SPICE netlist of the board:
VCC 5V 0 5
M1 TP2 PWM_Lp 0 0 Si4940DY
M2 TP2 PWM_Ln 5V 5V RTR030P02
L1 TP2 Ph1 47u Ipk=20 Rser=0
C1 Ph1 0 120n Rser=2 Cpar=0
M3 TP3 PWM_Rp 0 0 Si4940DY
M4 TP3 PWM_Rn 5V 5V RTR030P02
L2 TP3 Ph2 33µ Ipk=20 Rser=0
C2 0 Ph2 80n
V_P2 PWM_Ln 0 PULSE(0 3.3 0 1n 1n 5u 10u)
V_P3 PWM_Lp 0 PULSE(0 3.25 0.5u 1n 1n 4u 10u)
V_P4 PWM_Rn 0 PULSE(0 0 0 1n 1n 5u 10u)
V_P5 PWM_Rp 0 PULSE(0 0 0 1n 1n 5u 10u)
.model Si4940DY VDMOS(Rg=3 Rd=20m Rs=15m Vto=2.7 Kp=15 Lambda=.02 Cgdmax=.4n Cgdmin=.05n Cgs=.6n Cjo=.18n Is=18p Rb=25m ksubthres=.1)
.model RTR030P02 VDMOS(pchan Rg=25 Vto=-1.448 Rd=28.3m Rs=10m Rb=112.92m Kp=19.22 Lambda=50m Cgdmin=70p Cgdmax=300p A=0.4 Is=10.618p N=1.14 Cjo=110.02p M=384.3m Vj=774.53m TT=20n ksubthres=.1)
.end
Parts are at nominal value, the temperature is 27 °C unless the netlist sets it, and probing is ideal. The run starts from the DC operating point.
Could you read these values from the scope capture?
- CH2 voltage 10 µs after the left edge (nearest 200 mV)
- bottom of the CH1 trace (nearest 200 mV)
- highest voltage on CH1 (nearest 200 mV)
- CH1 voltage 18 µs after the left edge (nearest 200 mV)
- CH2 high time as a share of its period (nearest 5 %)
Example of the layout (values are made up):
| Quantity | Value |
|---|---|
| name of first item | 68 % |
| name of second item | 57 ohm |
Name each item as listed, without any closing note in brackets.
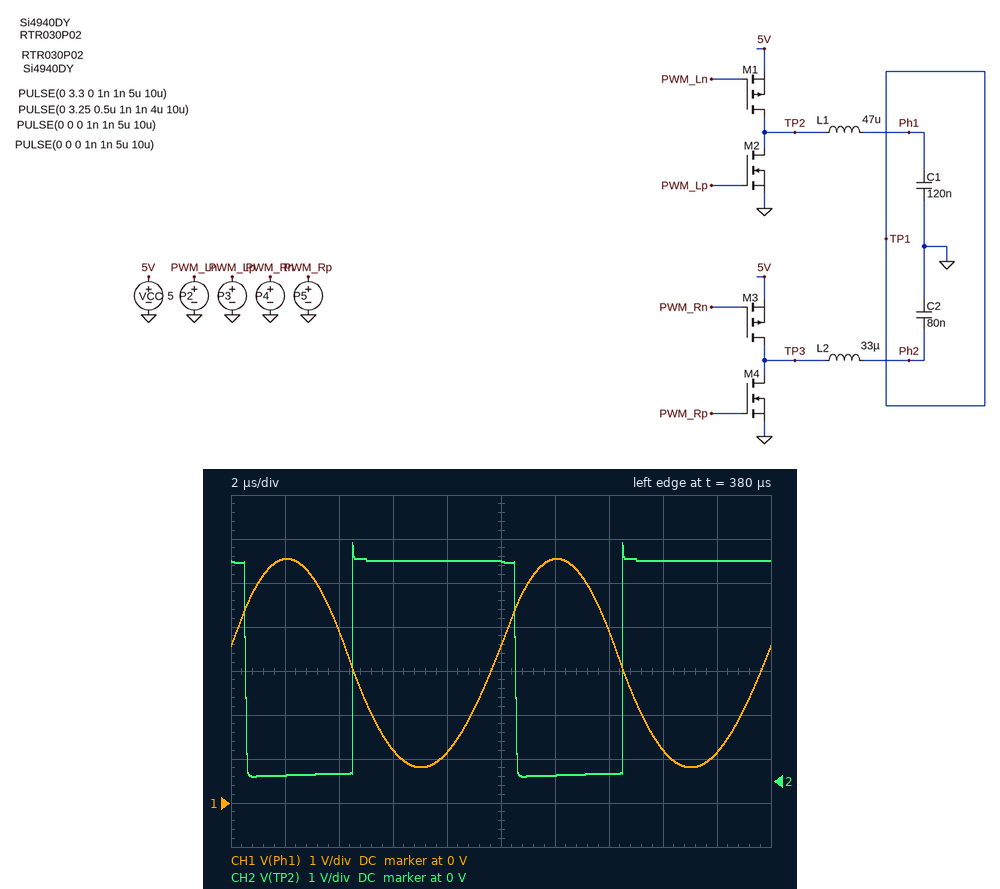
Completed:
| Quantity | Value |
|---|---|
| CH2 voltage 10 µs after the left edge | 5.0 V |
| bottom of the CH1 trace | 800 mV |
| highest voltage on CH1 | 5.6 V |
| CH1 voltage 18 µs after the left edge | 1.2 V |
| CH2 high time as a share of its period | 60 % |
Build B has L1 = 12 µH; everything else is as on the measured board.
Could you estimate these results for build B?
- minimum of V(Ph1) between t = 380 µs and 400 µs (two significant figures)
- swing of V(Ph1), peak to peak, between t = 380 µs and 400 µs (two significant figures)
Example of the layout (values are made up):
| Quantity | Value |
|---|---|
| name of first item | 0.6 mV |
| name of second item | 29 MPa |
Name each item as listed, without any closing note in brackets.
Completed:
| Quantity | Value |
|---|---|
| minimum of V(Ph1) between t = 380 µs and 400 µs | -3.1 V |
| swing of V(Ph1), peak to peak, between t = 380 µs and 400 µs | 13 V |
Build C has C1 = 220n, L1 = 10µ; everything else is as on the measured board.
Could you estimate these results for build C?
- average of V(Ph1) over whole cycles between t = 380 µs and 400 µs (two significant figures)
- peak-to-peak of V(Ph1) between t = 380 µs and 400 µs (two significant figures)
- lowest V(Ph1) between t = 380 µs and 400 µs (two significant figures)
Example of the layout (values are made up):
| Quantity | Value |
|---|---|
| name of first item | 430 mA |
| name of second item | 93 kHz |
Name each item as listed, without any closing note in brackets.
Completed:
| Quantity | Value |
|---|---|
| average of V(Ph1) over whole cycles between t = 380 µs and 400 µs | 3.2 V |
| peak-to-peak of V(Ph1) between t = 380 µs and 400 µs | 18 V |
| lowest V(Ph1) between t = 380 µs and 400 µs | -6.3 V |
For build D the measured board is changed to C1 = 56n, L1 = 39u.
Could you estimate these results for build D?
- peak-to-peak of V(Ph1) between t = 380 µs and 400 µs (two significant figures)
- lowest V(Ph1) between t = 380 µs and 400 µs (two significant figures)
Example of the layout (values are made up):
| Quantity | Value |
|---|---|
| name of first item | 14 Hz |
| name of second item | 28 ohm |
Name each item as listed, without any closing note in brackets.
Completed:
| Quantity | Value |
|---|---|
| peak-to-peak of V(Ph1) between t = 380 µs and 400 µs | 38 V |
| lowest V(Ph1) between t = 380 µs and 400 µs | -16 V |
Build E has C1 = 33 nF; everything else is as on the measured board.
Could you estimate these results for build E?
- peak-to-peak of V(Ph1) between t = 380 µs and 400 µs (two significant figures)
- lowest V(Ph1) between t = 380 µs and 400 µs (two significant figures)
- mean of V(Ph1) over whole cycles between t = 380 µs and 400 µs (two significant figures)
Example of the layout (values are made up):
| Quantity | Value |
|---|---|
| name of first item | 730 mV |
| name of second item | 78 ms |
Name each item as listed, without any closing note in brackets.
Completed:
| Quantity | Value |
|---|---|
| peak-to-peak of V(Ph1) between t = 380 µs and 400 µs | 15 V |
| lowest V(Ph1) between t = 380 µs and 400 µs | -4.0 V |
| mean of V(Ph1) over whole cycles between t = 380 µs and 400 µs | 3.1 V |
